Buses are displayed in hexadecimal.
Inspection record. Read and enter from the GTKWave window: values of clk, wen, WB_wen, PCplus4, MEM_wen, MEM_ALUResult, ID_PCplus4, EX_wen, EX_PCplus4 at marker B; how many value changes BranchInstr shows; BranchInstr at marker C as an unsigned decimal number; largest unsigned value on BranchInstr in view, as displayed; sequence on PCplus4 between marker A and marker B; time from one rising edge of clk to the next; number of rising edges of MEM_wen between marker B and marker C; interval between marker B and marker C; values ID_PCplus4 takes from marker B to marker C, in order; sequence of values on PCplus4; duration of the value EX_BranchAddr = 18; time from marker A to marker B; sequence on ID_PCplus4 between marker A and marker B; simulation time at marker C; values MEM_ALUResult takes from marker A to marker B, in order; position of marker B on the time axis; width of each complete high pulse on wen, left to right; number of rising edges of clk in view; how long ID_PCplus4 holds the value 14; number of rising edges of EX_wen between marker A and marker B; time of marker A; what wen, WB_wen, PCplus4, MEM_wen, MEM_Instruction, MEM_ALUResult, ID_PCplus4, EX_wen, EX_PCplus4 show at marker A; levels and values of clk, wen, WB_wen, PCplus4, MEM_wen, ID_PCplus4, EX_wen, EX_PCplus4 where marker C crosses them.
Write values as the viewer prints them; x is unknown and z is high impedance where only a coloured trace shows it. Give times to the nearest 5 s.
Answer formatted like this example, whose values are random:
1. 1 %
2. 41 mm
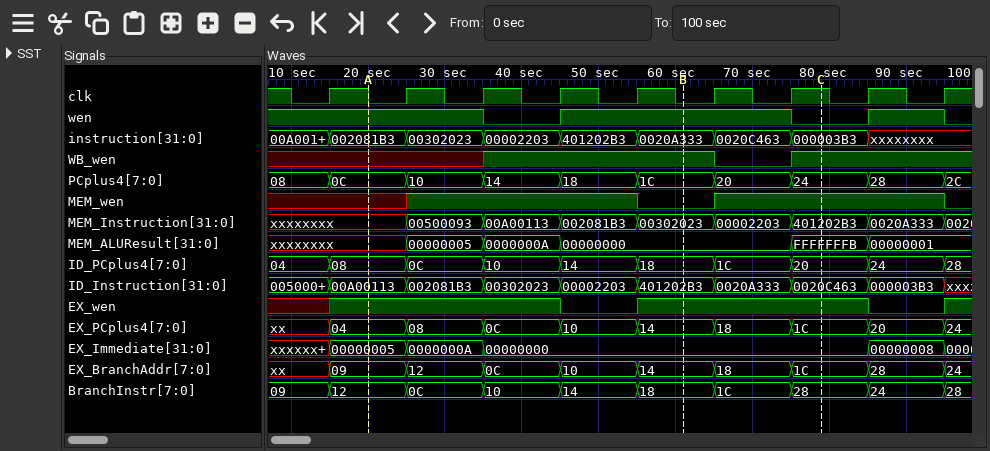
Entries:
1. clk=0, wen=1, WB_wen=1, PCplus4=1C, MEM_wen=0, MEM_ALUResult=00000000, ID_PCplus4=18, EX_wen=1, EX_PCplus4=14
2. 9
3. 40
4. 28
5. 0C, 10, 14, 18, 1C
6. 10 s
7. 1
8. 20 s
9. 18, 1C, 20
10. 08, 0C, 10, 14, 18, 1C, 20, 24, 28, 2C
11. 10 s
12. 40 s
13. 08, 0C, 10, 14, 18
14. 80 s
15. xxxxxxxx, 00000005, 0000000A, 00000000
16. 60 s
17. 30 s, 10 s
18. 9
19. 10 s
20. 1
21. 20 s
22. wen=1, WB_wen=x, PCplus4=0C, MEM_wen=x, MEM_Instruction=xxxxxxxx, MEM_ALUResult=xxxxxxxx, ID_PCplus4=08, EX_wen=1, EX_PCplus4=04
23. clk=1, wen=0, WB_wen=1, PCplus4=24, MEM_wen=1, ID_PCplus4=20, EX_wen=1, EX_PCplus4=1C
